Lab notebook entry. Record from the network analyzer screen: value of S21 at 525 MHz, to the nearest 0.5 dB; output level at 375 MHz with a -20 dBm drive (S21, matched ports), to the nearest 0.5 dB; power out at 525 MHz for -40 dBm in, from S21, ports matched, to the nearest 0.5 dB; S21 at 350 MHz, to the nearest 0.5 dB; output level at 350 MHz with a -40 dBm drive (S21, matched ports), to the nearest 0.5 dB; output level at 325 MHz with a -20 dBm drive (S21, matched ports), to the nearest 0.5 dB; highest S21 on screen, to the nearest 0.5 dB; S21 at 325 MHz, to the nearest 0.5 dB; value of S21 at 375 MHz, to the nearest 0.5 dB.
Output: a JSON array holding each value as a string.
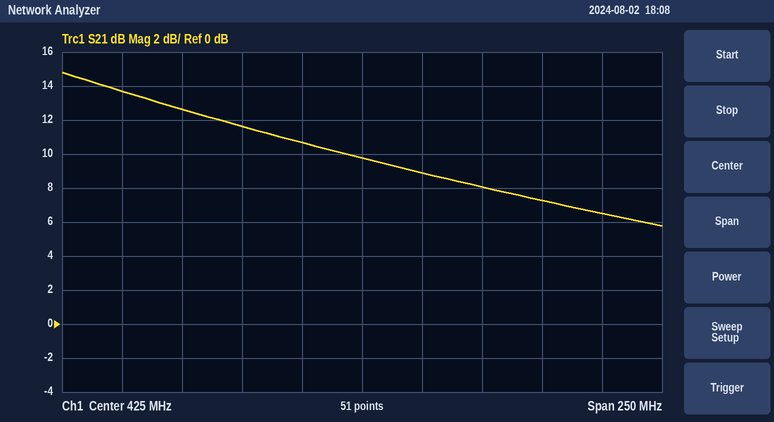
["6.5 dB", "-8.5 dBm", "-33.5 dBm", "12.5 dB", "-27.5 dBm", "-6.5 dBm", "15.0 dB", "13.5 dB", "11.5 dB"]
